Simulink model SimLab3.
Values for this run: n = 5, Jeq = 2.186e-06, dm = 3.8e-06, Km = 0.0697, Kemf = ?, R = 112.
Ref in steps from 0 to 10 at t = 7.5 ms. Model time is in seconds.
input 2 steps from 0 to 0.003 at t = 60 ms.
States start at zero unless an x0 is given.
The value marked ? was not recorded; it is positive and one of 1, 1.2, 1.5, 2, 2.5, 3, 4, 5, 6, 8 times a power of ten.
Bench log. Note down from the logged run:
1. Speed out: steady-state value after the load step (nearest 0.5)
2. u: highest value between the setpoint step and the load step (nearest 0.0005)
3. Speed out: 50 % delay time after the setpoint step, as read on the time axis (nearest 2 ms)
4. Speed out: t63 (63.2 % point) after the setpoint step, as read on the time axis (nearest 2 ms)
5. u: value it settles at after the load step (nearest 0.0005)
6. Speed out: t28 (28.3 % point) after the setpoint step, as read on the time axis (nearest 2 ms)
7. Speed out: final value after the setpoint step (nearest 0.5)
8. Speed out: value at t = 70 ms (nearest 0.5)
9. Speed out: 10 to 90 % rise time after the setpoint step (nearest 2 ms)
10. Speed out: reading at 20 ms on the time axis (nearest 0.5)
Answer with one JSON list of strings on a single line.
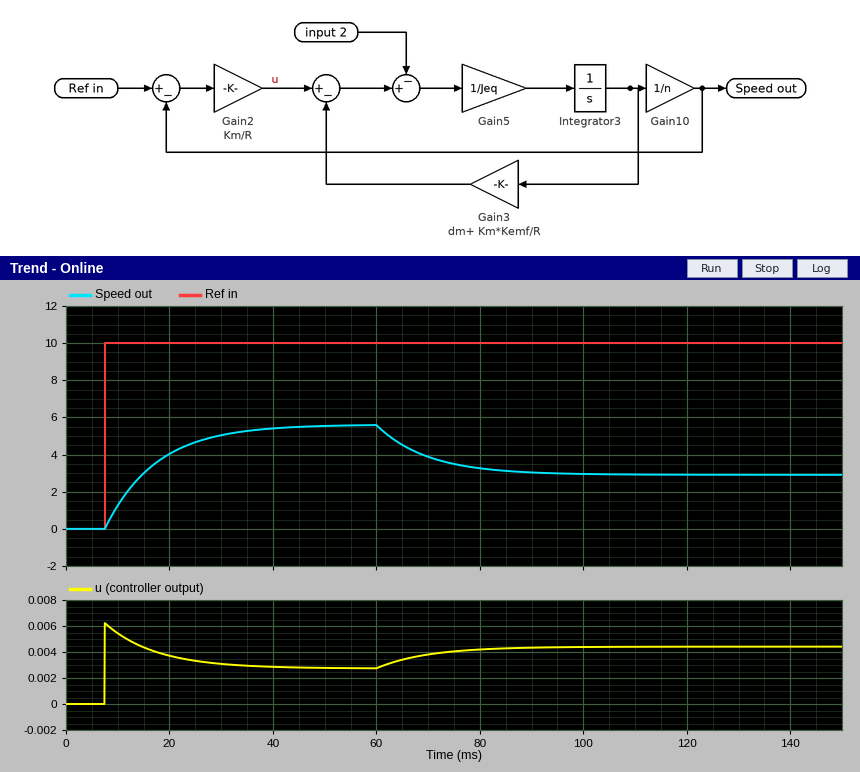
["3.0", "0.0060", "14 ms", "18 ms", "0.0045", "10 ms", "5.5", "4.0", "22 ms", "4.0"]
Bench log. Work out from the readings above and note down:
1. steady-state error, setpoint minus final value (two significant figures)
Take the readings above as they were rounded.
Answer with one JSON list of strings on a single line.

["4.5"]
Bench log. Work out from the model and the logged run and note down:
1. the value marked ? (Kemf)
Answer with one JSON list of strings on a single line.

["0.15"]
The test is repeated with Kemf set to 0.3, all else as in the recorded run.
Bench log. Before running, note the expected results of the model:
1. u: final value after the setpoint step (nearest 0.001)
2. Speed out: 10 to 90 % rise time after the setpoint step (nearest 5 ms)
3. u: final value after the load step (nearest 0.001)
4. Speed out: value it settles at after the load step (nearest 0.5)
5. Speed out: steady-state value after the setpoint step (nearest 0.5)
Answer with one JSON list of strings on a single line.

["0.004", "15 ms", "0.005", "2.0", "4.0"]
